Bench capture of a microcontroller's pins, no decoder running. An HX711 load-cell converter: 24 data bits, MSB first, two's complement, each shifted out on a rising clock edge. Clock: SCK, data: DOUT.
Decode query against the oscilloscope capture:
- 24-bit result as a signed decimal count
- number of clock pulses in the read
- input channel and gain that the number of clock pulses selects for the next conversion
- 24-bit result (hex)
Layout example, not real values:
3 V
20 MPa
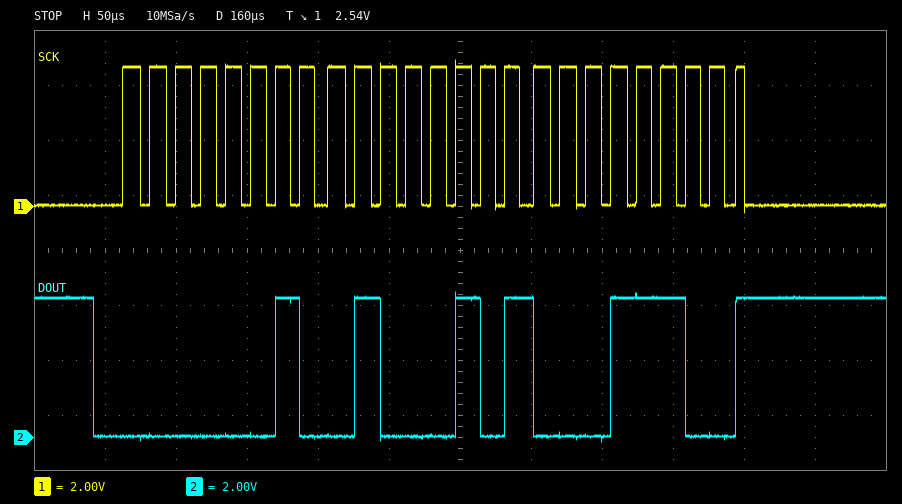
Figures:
148764
25
channel A, gain 128
0x02451C
